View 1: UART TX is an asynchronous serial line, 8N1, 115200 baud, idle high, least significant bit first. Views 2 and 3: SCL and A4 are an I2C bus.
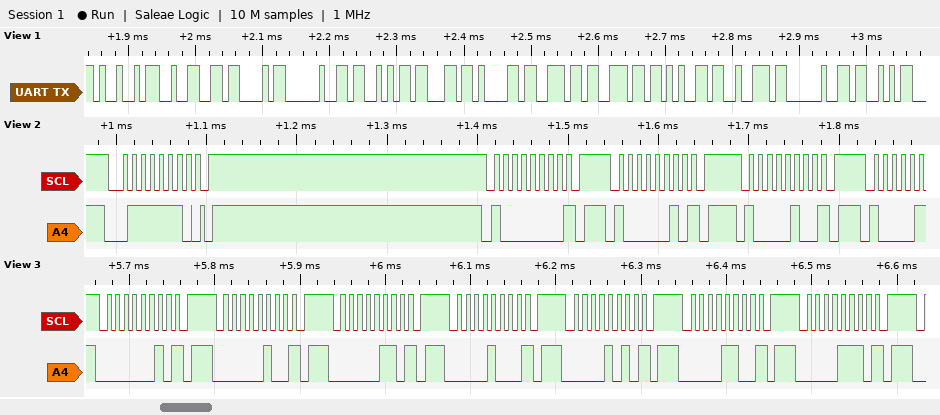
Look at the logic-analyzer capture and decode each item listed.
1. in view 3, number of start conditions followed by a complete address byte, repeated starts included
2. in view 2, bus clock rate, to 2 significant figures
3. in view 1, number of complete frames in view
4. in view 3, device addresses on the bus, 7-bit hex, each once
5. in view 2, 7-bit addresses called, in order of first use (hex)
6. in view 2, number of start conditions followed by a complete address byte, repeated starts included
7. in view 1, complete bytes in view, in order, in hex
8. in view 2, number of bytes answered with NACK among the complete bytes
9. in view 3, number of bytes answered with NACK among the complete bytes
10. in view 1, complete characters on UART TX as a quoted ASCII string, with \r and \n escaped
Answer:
7
100 kHz
13
0x01 0x02 0x03 0x04 0x05 0x06 0x07
0x3F 0x40 0x41 0x42
4
49 32 43 20 53 63 61 6E 6E 65 72 20 53
3
7
"I2C Scanner S"
